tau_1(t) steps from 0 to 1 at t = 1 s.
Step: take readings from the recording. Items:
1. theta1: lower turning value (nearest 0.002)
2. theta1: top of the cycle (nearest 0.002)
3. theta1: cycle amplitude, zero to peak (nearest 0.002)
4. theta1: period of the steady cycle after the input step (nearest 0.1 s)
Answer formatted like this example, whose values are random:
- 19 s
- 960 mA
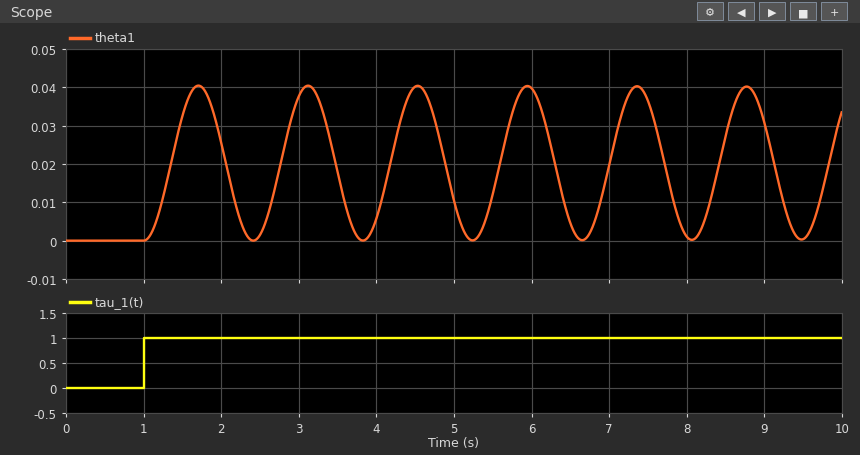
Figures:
- 0.000
- 0.040
- 0.020
- 1.4 s
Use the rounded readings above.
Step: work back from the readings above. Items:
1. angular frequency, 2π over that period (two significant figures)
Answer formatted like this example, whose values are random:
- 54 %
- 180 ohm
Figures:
- 4.5 rad/s
